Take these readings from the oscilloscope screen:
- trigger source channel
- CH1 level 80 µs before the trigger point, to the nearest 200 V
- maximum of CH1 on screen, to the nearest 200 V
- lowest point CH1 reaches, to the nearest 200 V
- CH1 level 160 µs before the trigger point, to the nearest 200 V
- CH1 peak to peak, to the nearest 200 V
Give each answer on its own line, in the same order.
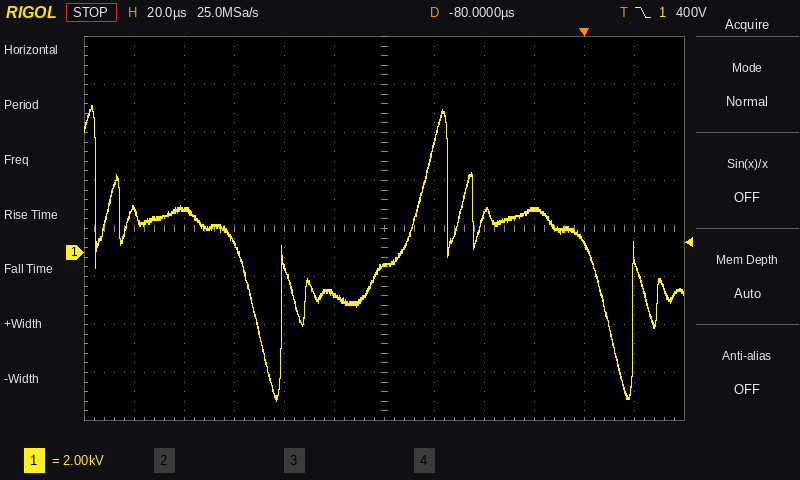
CH1
-600 V
6.2 kV
-6.2 kV
1.8 kV
12.4 kV
